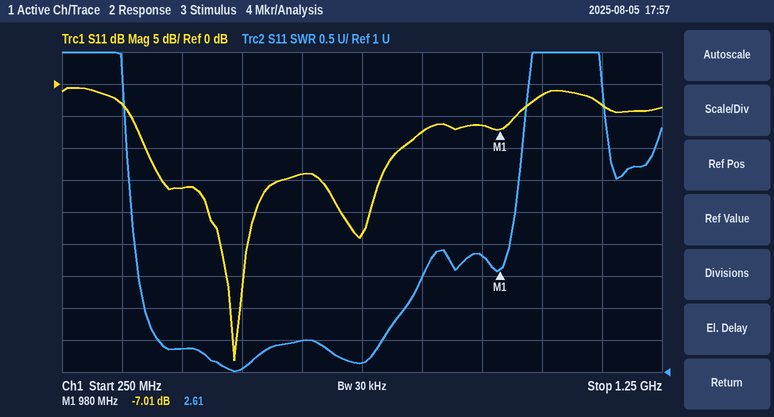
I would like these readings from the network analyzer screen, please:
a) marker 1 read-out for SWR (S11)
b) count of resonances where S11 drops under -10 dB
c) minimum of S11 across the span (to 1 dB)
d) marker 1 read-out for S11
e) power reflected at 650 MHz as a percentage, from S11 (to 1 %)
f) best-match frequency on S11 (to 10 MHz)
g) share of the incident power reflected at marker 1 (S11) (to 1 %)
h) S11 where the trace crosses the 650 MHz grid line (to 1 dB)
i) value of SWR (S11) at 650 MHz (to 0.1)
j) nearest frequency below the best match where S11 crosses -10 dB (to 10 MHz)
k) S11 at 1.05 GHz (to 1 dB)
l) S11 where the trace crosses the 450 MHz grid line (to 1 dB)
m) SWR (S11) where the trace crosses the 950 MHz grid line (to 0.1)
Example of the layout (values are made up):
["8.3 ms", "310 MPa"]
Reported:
["2.61", "2", "-43 dB", "-7.01 dB", "4 %", "540 MHz", "20 %", "-14 dB", "1.5", "390 MHz", "-2 dB", "-16 dB", "2.8"]
